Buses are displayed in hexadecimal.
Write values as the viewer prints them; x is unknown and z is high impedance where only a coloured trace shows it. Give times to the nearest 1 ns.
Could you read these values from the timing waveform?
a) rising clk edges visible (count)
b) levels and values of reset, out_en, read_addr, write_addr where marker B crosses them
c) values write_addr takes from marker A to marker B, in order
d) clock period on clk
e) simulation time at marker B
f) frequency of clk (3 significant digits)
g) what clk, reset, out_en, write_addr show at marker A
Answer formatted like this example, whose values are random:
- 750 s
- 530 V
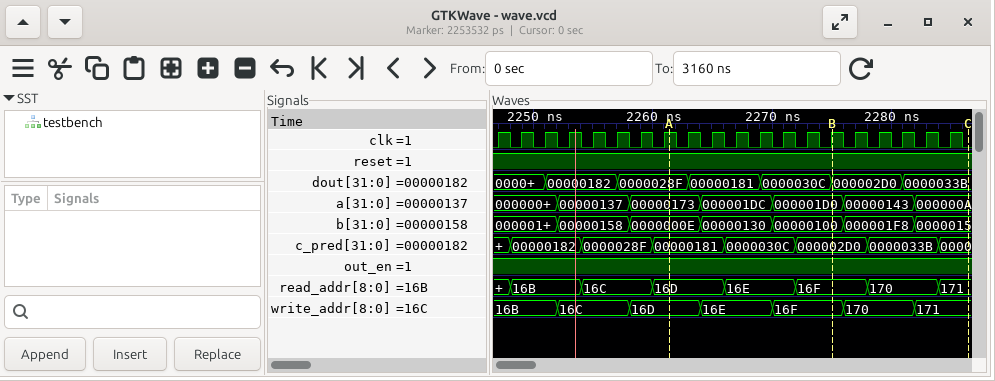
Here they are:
- 20
- reset=1, out_en=1, read_addr=16F, write_addr=16F
- 16D, 16E, 16F
- 2 ns
- 2275 ns
- 500 MHz
- clk=1, reset=1, out_en=1, write_addr=16D
